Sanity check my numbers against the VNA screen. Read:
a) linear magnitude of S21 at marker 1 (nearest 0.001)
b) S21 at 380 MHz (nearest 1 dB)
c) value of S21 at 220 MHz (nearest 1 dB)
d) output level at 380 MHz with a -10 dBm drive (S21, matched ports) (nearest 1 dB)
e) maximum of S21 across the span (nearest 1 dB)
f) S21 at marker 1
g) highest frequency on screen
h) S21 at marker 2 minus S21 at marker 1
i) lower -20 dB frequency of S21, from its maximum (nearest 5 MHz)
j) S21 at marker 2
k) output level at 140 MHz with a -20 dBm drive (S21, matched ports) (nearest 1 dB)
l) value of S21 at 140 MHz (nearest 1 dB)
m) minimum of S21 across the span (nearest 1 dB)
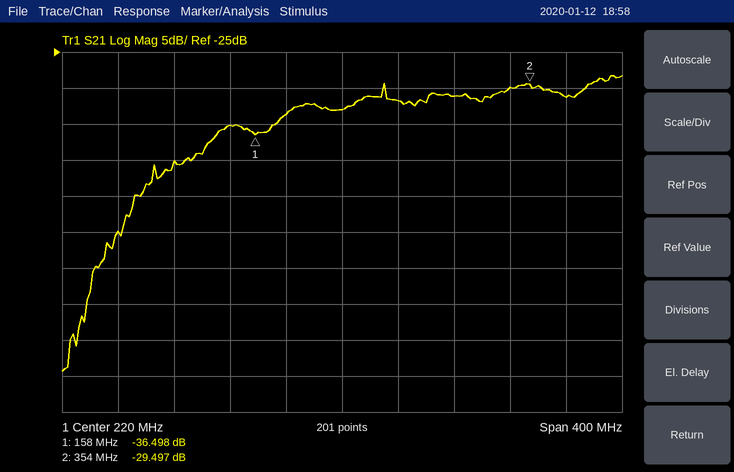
0.015
-31 dB
-33 dB
-41 dBm
-28 dB
-36.498 dB
420 MHz
7.001 dB
65 MHz
-29.497 dB
-55 dBm
-35 dB
-69 dB
